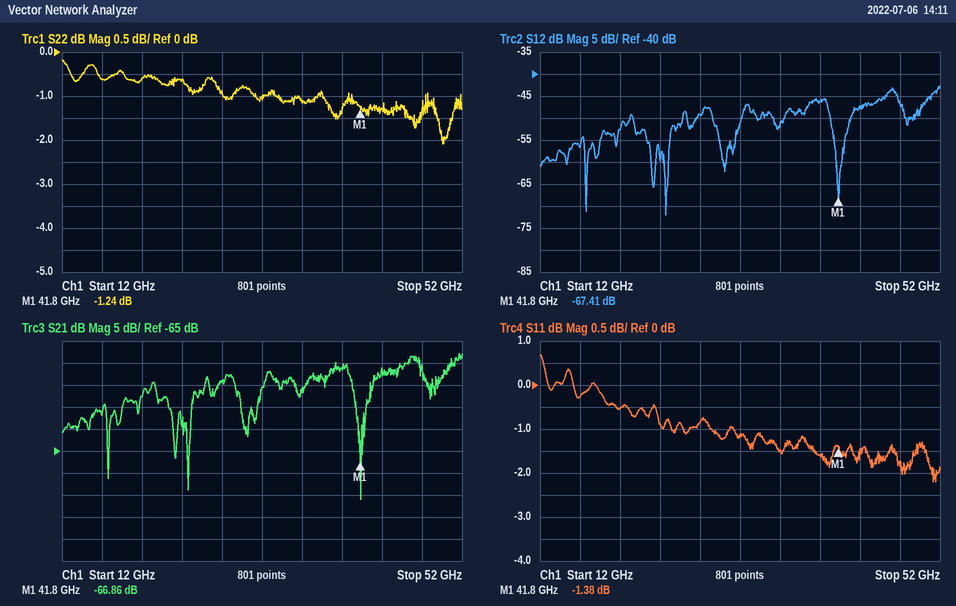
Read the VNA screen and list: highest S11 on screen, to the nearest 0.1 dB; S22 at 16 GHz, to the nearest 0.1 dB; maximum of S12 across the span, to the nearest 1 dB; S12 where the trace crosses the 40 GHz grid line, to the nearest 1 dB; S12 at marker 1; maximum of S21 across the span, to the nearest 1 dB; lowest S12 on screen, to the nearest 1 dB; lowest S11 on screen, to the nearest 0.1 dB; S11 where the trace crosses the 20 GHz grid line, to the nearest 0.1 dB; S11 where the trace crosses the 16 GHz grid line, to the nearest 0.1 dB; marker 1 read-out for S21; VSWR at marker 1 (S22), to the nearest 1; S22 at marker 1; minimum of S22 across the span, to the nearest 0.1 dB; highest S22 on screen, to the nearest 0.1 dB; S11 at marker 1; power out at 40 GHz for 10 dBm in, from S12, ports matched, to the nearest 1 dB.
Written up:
0.7 dB
-0.6 dB
-43 dB
-46 dB
-67.41 dB
-43 dB
-72 dB
-2.2 dB
-0.5 dB
-0.3 dB
-66.86 dB
14
-1.24 dB
-2.1 dB
-0.2 dB
-1.38 dB
-36 dBm
